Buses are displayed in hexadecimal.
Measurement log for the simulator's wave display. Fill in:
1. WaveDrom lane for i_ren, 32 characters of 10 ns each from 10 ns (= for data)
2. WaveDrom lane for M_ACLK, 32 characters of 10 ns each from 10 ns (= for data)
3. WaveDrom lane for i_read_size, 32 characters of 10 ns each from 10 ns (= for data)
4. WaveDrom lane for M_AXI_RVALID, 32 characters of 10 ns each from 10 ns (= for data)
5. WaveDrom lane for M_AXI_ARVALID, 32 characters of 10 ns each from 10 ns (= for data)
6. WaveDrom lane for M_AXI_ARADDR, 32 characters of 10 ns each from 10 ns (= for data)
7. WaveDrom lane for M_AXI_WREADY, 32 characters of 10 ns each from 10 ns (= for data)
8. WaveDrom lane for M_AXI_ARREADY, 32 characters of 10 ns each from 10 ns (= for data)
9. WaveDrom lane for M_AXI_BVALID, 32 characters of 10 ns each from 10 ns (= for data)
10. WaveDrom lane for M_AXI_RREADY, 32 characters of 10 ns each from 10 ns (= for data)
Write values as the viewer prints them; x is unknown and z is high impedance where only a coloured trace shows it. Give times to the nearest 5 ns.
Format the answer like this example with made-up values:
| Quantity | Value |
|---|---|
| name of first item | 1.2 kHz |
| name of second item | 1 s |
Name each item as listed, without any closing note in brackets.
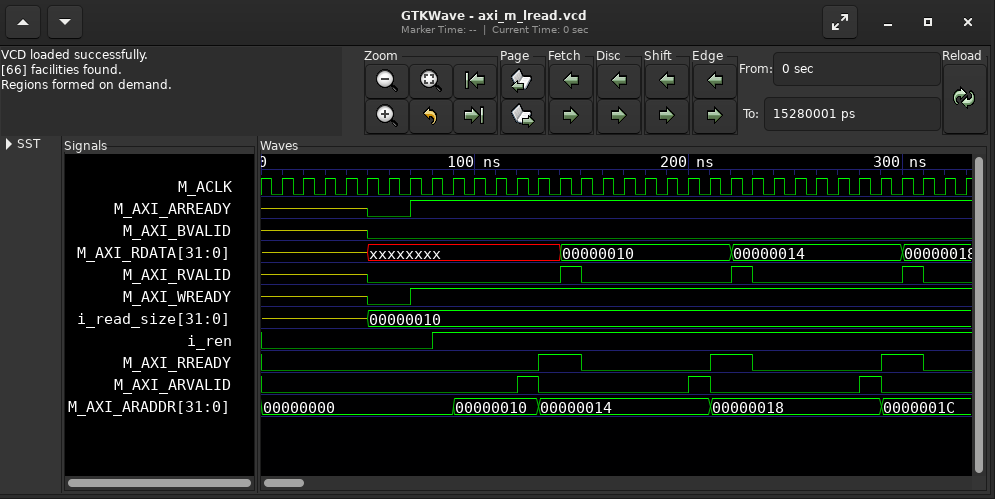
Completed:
| Quantity | Value |
|---|---|
| WaveDrom lane for i_ren, 32 characters of 10 ns each from 10 ns | {name: 'i_ren', wave: '0......1........................'} |
| WaveDrom lane for M_ACLK, 32 characters of 10 ns each from 10 ns | {name: 'M_ACLK', wave: 'p...............................'} |
| WaveDrom lane for i_read_size, 32 characters of 10 ns each from 10 ns | {name: 'i_read_size', wave: 'z...=...........................', data: '00000010'} |
| WaveDrom lane for M_AXI_RVALID, 32 characters of 10 ns each from 10 ns | {name: 'M_AXI_RVALID', wave: 'z...0........10......10......10.'} |
| WaveDrom lane for M_AXI_ARVALID, 32 characters of 10 ns each from 10 ns | {name: 'M_AXI_ARVALID', wave: '0..........10......10......10...'} |
| WaveDrom lane for M_AXI_ARADDR, 32 characters of 10 ns each from 10 ns | {name: 'M_AXI_ARADDR', wave: '=.......=...=.......=.......=...', data: '00000000 00000010 00000014 00000018 0000001C'} |
| WaveDrom lane for M_AXI_WREADY, 32 characters of 10 ns each from 10 ns | {name: 'M_AXI_WREADY', wave: 'z...0.1.........................'} |
| WaveDrom lane for M_AXI_ARREADY, 32 characters of 10 ns each from 10 ns | {name: 'M_AXI_ARREADY', wave: 'z...0.1.........................'} |
| WaveDrom lane for M_AXI_BVALID, 32 characters of 10 ns each from 10 ns | {name: 'M_AXI_BVALID', wave: 'z...0...........................'} |
| WaveDrom lane for M_AXI_RREADY, 32 characters of 10 ns each from 10 ns | {name: 'M_AXI_RREADY', wave: '0...........1.0.....1.0.....1.0.'} |
